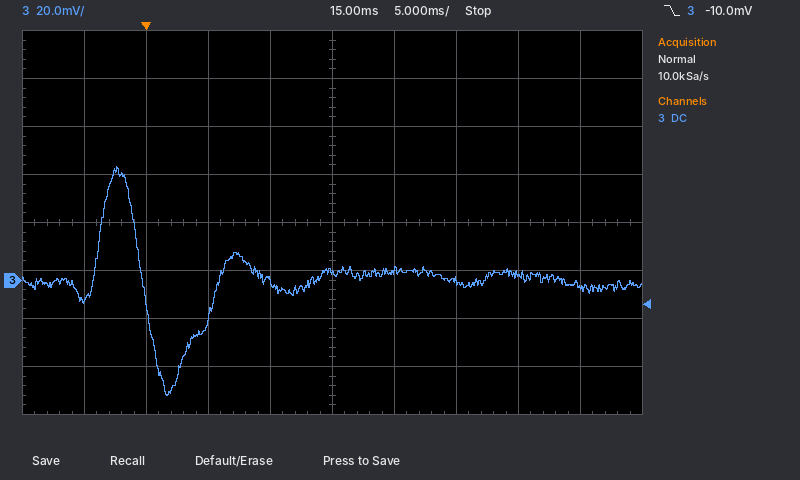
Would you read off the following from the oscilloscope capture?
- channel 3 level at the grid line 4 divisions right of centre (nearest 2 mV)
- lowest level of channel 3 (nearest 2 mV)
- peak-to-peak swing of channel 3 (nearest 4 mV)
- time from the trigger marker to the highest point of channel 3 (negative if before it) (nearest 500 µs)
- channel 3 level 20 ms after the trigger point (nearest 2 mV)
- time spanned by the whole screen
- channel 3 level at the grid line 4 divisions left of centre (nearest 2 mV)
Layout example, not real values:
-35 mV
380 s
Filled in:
-2 mV
-48 mV
96 mV
-2.5 ms
4 mV
50 ms
-8 mV
